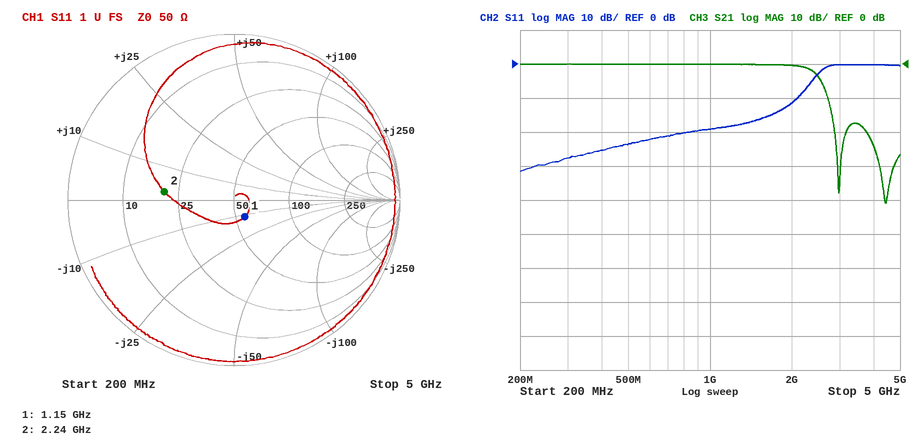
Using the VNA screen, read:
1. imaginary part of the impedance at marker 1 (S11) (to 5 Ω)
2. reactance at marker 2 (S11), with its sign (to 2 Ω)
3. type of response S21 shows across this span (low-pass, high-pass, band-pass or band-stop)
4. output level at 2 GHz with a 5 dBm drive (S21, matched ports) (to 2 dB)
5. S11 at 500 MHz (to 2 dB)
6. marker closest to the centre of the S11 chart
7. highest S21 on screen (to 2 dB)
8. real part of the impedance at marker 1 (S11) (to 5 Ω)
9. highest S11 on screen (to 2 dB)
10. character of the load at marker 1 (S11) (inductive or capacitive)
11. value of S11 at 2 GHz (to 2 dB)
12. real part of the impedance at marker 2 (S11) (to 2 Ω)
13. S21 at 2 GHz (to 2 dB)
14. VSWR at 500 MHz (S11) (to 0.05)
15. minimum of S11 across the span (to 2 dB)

-10 Ω
+2 Ω
low-pass
4 dBm
-24 dB
marker 1
0 dB
55 Ω
0 dB
capacitive
-12 dB
20 Ω
0 dB
1.15
-32 dB
